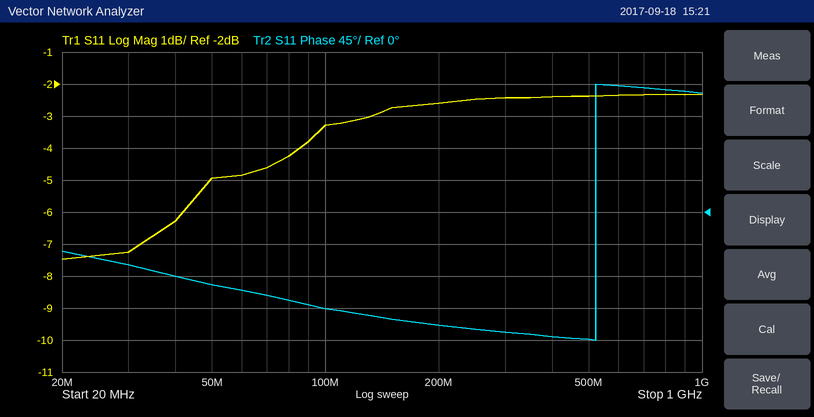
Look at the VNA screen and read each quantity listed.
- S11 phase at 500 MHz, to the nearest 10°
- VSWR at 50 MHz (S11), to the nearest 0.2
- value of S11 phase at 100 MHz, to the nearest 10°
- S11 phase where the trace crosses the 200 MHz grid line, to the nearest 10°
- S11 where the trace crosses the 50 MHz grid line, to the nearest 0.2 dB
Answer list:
-180°
3.6
-140°
-160°
-5.0 dB
